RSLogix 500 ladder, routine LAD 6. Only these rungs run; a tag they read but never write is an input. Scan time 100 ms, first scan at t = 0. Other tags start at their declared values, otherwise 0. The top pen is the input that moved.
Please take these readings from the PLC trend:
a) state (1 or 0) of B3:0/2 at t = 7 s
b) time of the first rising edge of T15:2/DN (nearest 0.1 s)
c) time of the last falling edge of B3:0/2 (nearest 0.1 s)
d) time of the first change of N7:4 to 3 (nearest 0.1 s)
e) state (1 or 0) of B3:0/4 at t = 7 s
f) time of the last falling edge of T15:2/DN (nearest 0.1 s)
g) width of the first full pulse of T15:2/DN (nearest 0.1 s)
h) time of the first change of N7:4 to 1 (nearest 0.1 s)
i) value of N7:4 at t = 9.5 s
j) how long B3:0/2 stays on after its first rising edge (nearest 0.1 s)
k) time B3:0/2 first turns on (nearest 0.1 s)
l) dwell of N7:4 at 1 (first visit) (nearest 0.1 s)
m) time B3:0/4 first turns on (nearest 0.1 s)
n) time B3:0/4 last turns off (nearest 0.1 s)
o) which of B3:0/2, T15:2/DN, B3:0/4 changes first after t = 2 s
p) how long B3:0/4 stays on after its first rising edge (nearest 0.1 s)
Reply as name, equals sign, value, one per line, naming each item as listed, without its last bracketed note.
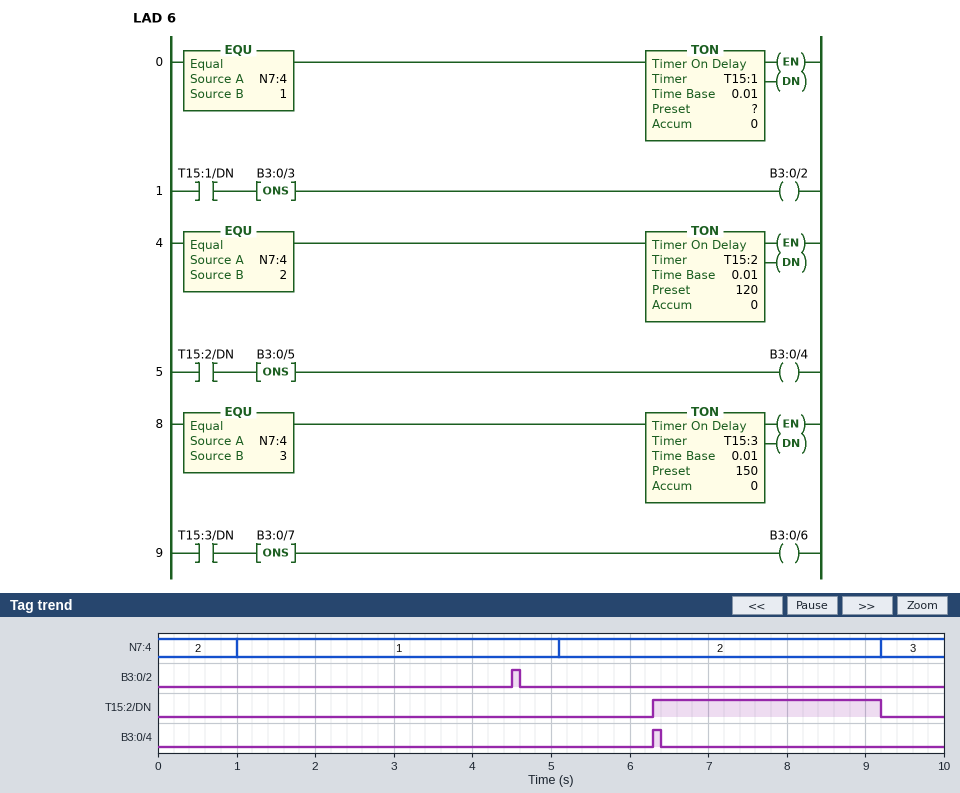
state (1 or 0) of B3:0/2 at t = 7 s = 0
time of the first rising edge of T15:2/DN = 6.3 s
time of the last falling edge of B3:0/2 = 4.6 s
time of the first change of N7:4 to 3 = 9.2 s
state (1 or 0) of B3:0/4 at t = 7 s = 0
time of the last falling edge of T15:2/DN = 9.2 s
width of the first full pulse of T15:2/DN = 2.9 s
time of the first change of N7:4 to 1 = 1.0 s
value of N7:4 at t = 9.5 s = 3
how long B3:0/2 stays on after its first rising edge = 0.1 s
time B3:0/2 first turns on = 4.5 s
dwell of N7:4 at 1 (first visit) = 4.1 s
time B3:0/4 first turns on = 6.3 s
time B3:0/4 last turns off = 6.4 s
which of B3:0/2, T15:2/DN, B3:0/4 changes first after t = 2 s = B3:0/2
how long B3:0/4 stays on after its first rising edge = 0.1 s
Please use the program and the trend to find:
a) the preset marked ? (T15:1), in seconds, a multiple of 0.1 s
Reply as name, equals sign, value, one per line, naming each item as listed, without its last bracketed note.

the preset marked ? (T15:1), in seconds, a multiple of 0.1 s = 3.5 s
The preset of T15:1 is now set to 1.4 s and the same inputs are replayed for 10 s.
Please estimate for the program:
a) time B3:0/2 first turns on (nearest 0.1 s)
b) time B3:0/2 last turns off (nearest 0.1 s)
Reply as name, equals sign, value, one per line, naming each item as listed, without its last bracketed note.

time B3:0/2 first turns on = 2.4 s
time B3:0/2 last turns off = 2.5 s
